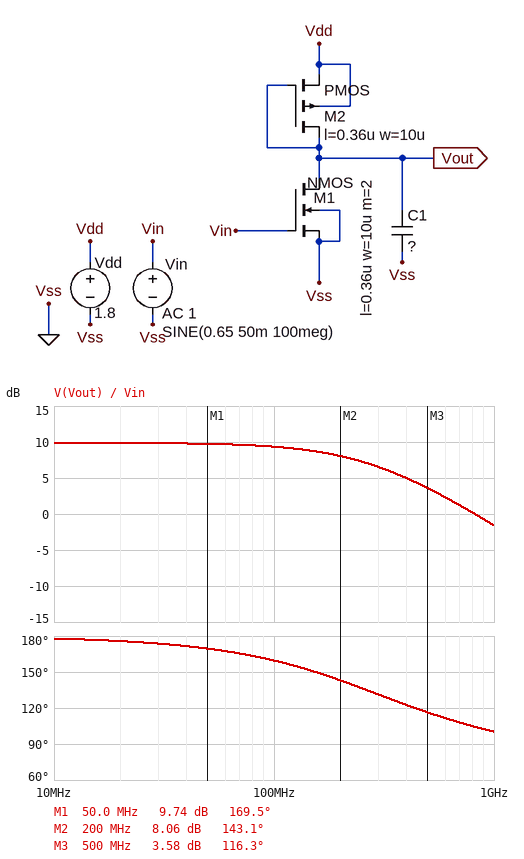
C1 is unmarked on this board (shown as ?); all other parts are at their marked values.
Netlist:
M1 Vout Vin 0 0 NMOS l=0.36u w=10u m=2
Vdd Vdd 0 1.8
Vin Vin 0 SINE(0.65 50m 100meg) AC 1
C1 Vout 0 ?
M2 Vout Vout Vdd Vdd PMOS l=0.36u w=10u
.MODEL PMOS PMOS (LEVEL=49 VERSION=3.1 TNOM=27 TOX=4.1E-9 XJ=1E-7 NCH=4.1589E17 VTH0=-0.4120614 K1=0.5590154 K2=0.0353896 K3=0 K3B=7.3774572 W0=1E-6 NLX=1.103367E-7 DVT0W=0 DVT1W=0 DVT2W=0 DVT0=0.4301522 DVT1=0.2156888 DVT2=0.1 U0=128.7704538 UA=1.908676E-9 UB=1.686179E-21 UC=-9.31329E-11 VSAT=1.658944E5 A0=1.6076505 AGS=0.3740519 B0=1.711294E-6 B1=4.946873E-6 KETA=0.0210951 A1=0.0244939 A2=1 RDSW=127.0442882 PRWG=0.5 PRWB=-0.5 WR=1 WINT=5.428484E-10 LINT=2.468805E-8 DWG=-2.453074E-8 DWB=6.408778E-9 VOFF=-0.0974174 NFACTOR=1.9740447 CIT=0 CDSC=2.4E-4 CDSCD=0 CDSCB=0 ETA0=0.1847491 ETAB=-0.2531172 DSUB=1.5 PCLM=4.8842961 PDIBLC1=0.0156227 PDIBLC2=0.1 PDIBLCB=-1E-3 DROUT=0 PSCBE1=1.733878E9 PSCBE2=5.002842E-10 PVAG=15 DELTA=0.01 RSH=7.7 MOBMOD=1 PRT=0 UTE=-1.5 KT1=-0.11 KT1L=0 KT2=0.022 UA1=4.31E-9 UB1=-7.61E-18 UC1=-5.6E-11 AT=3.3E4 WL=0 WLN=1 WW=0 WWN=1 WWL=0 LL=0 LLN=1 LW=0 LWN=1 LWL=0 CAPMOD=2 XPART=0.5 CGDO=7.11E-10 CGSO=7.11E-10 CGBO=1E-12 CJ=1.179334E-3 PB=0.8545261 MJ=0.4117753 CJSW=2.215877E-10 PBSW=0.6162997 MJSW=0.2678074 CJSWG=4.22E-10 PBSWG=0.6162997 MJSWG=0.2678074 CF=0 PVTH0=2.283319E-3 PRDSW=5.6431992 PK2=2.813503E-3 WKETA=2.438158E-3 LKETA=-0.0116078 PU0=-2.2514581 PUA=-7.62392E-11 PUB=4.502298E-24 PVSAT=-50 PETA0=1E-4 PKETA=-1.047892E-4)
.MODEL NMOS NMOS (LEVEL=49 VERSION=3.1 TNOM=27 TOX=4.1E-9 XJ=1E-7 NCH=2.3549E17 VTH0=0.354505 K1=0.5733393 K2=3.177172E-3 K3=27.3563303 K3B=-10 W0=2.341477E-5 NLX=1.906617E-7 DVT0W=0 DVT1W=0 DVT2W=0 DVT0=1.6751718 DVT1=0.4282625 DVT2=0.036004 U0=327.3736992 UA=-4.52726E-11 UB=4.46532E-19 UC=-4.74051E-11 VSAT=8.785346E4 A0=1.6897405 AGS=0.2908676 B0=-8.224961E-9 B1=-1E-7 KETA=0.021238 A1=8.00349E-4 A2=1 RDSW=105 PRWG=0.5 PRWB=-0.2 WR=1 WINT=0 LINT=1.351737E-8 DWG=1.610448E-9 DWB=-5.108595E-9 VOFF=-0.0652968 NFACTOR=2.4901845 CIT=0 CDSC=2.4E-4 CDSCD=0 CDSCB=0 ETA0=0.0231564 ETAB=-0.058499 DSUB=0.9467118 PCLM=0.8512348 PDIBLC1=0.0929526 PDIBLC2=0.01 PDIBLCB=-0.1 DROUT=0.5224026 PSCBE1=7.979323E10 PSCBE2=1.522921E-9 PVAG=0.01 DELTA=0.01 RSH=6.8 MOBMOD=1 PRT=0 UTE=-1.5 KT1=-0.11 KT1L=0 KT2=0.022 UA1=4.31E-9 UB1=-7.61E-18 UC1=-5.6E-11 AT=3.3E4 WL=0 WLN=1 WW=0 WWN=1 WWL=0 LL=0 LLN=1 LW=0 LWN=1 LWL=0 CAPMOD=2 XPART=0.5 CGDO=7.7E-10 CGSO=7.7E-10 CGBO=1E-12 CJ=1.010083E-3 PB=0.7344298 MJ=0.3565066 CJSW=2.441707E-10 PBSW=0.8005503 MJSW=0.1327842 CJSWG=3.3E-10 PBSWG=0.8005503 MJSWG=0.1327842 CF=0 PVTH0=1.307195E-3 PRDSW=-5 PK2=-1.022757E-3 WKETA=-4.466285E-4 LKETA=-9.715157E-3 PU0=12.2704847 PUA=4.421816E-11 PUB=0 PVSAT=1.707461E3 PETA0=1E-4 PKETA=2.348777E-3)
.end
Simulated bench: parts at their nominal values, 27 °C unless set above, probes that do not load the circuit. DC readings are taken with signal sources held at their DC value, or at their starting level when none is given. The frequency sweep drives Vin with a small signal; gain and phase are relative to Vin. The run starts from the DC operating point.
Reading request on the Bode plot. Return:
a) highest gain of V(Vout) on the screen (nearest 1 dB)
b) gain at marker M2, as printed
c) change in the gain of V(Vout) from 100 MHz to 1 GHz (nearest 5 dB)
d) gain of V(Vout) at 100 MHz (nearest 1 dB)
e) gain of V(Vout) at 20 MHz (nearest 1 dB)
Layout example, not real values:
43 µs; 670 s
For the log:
10 dB; 8.06 dB; -10 dB; 9 dB; 10 dB
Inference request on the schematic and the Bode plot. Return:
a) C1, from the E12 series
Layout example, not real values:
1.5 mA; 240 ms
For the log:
390 fF
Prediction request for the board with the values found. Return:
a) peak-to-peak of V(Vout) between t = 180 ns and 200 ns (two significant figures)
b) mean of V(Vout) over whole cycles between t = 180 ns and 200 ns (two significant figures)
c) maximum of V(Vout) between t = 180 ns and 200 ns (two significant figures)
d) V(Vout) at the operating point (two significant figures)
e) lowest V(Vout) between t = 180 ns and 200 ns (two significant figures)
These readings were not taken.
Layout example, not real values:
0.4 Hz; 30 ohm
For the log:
290 mV; 850 mV; 990 mV; 860 mV; 700 mV
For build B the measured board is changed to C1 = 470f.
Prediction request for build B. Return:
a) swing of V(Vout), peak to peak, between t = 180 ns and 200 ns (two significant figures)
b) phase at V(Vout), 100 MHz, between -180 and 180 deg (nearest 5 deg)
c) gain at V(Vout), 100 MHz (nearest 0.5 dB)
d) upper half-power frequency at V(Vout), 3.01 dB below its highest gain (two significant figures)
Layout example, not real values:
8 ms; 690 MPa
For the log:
280 mV; 155 deg; 9.0 dB; 230 MHz
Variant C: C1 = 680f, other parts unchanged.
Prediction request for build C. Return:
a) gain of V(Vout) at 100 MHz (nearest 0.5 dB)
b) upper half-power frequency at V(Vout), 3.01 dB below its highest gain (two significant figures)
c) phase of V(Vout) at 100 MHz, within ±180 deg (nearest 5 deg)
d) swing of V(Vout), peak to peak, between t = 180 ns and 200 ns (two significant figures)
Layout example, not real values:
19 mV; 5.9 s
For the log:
8.5 dB; 170 MHz; 150 deg; 260 mV
